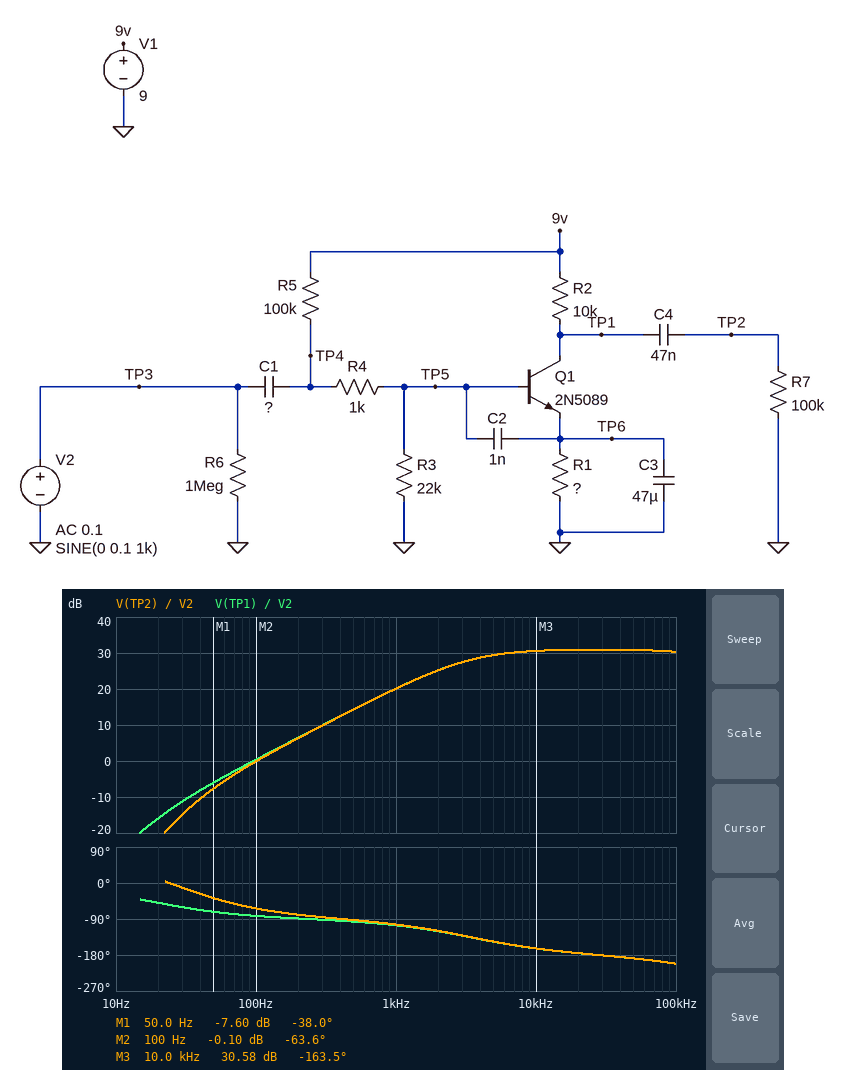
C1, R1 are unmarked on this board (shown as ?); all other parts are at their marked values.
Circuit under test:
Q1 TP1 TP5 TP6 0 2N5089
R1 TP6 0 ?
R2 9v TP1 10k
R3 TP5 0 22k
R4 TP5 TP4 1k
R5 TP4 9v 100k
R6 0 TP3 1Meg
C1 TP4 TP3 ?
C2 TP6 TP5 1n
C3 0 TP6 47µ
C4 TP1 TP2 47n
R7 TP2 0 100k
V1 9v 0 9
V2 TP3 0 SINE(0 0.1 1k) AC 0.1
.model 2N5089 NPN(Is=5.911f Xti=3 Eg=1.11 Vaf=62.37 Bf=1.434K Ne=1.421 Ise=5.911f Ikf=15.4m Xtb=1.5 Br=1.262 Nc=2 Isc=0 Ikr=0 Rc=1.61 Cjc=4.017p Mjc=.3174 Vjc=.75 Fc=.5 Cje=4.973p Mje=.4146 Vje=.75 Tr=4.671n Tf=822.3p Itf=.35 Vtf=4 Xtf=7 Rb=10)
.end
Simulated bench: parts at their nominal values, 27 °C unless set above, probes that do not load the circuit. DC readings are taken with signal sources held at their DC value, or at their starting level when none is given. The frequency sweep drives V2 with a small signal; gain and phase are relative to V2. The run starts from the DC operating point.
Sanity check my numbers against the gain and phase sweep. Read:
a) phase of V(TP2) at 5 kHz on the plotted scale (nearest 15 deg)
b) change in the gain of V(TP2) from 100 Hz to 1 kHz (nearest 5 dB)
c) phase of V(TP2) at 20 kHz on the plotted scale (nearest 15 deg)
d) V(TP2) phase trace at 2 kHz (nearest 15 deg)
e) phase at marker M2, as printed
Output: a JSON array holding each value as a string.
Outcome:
["-150 deg", "20 dB", "-180 deg", "-120 deg", "-63.6 deg"]
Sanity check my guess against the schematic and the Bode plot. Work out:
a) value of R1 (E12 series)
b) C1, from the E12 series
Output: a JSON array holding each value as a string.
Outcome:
["5.6 kΩ", "1.8 nF"]
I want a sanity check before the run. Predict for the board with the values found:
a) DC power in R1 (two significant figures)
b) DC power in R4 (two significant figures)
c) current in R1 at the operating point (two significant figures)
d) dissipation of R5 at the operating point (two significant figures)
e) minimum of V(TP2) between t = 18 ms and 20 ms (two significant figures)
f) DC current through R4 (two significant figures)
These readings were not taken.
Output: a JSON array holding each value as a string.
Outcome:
["170 µW", "5.4 µW", "180 µA", "540 µW", "-1.1 V", "73 µA"]
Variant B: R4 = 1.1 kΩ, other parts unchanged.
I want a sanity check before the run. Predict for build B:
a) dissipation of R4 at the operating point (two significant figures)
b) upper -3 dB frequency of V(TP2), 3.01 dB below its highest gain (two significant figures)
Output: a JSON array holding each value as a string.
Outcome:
["5.9 µW", "220 kHz"]
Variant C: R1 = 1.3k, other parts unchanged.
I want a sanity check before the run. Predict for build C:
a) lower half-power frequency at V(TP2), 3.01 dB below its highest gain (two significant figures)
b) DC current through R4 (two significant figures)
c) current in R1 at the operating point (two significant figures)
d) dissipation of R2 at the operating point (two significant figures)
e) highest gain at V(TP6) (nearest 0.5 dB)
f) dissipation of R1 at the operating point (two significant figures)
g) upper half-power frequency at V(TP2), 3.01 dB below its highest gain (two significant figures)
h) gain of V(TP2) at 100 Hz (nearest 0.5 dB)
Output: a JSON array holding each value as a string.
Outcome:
["3.6 kHz", "73 µA", "720 µA", "5.1 mW", "-39.5 dB", "670 µW", "180 kHz", "7.5 dB"]
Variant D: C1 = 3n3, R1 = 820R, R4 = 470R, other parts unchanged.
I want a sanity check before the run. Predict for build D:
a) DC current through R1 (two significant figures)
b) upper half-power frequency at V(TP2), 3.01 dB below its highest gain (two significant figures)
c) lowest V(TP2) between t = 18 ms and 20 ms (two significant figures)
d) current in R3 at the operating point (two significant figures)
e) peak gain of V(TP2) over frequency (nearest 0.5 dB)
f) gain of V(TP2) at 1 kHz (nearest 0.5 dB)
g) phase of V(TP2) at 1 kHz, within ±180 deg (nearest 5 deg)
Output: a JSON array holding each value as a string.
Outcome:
["840 µA", "2.1 MHz", "-3.6 mV", "61 µA", "10.0 dB", "-28.5 dB", "-90 deg"]
